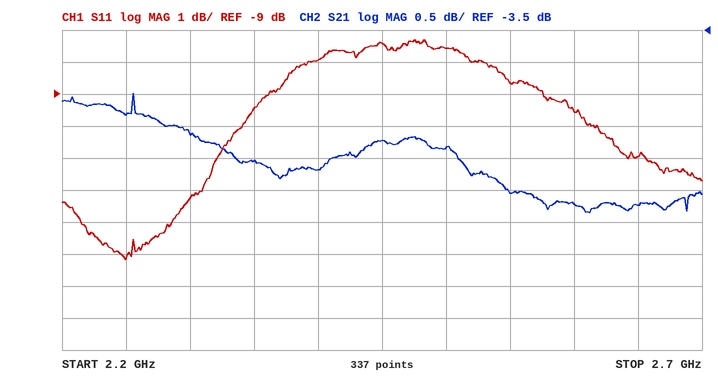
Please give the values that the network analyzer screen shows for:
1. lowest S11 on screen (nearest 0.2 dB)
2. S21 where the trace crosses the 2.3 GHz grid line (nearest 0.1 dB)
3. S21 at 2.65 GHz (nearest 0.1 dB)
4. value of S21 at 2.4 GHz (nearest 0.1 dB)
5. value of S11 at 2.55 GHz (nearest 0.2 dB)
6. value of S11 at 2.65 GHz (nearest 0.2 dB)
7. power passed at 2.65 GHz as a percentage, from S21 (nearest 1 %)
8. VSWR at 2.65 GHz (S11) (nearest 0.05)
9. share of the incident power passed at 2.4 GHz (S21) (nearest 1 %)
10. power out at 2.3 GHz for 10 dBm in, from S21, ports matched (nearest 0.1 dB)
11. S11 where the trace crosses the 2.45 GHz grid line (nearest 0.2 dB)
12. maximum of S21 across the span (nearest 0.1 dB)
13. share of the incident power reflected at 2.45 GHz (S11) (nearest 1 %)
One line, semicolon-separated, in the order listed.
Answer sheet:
-14.2 dB; -5.1 dB; -6.2 dB; -5.7 dB; -8.6 dB; -11.0 dB; 24 %; 1.80; 27 %; 4.9 dBm; -7.4 dB; -4.5 dB; 18 %
